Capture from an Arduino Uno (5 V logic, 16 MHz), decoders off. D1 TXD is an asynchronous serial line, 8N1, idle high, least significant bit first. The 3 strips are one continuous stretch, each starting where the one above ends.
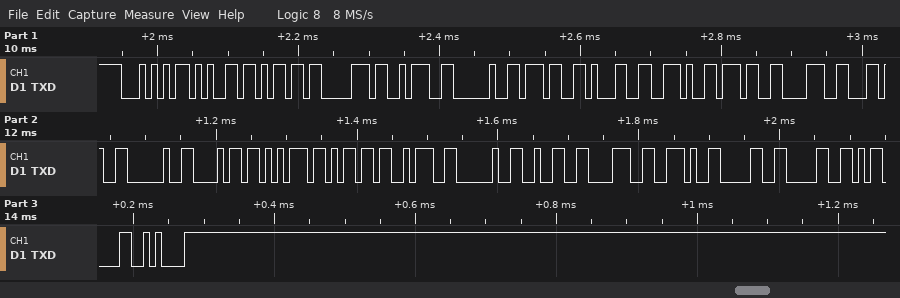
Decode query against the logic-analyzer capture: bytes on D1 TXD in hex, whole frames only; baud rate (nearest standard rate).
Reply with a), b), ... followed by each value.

a) 0x54 0x65 0x6D 0x70 0x3A 0x20 0x37 0x31 0x2E 0x37 0x38 0x2C 0x20 0x68 0x75 0x6D 0x3A 0x20 0x32 0x38 0x2E 0x30 0x30 0x0D 0x0A
b) 115200 baud
